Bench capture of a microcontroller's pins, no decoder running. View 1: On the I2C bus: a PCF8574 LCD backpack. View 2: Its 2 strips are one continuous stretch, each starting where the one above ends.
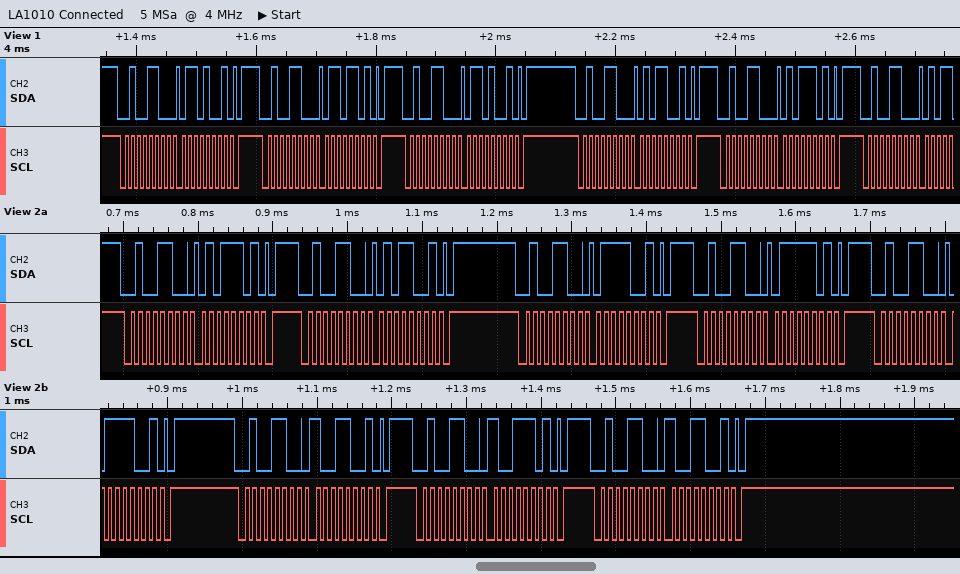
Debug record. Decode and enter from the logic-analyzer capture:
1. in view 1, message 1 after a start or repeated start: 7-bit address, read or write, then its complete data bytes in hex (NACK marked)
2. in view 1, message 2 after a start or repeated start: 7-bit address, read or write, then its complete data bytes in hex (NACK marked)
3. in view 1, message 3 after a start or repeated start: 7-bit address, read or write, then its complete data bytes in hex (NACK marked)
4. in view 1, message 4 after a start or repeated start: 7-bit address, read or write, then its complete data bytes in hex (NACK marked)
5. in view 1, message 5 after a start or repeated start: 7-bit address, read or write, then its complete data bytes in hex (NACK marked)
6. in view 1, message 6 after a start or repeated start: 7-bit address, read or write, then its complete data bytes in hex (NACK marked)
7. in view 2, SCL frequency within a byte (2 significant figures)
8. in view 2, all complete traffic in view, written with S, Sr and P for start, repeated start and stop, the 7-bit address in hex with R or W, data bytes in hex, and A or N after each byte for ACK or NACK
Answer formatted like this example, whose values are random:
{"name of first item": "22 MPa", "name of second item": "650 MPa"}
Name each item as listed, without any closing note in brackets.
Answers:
{"in view 1, message 1 after a start or repeated start: 7-bit address, read or write, then its complete data bytes in hex": "0x26 write: 69", "in view 1, message 2 after a start or repeated start: 7-bit address, read or write, then its complete data bytes in hex": "0x26 write: 6D", "in view 1, message 3 after a start or repeated start: 7-bit address, read or write, then its complete data bytes in hex": "0x26 write: 69", "in view 1, message 4 after a start or repeated start: 7-bit address, read or write, then its complete data bytes in hex": "0x26 write: 59", "in view 1, message 5 after a start or repeated start: 7-bit address, read or write, then its complete data bytes in hex": "0x26 write: 5D", "in view 1, message 6 after a start or repeated start: 7-bit address, read or write, then its complete data bytes in hex": "0x26 write", "in view 2, SCL frequency within a byte": "100 kHz", "in view 2, all complete traffic in view, written with S, Sr and P for start, repeated start and stop, the 7-bit address in hex with R or W, data bytes in hex, and A or N after each byte for ACK or NACK": "S 26W A 5D A P S 26W A 59 A P S 26W A 79 A P S 26W A 7D A P S 26W A 79 A P S 26W A 99 A P S 26W A 9D A P S 26W A 99 A P"}
